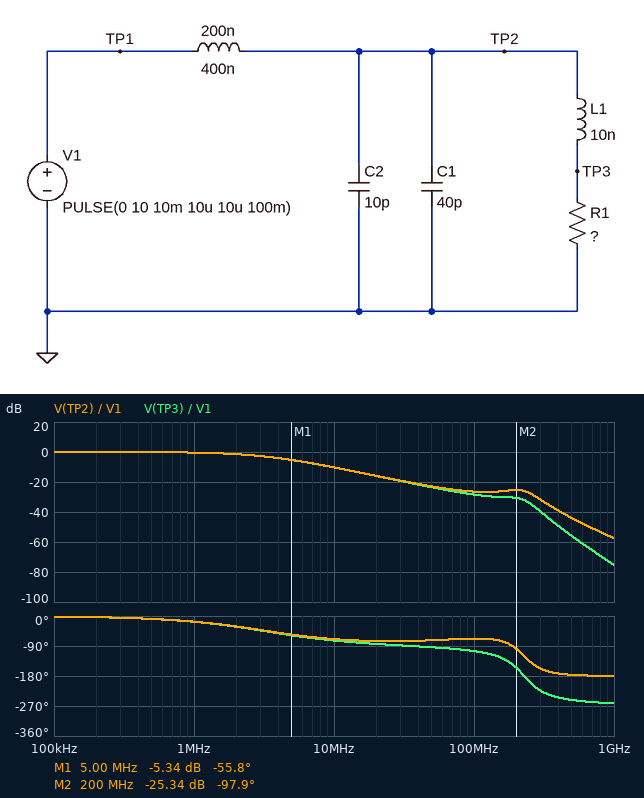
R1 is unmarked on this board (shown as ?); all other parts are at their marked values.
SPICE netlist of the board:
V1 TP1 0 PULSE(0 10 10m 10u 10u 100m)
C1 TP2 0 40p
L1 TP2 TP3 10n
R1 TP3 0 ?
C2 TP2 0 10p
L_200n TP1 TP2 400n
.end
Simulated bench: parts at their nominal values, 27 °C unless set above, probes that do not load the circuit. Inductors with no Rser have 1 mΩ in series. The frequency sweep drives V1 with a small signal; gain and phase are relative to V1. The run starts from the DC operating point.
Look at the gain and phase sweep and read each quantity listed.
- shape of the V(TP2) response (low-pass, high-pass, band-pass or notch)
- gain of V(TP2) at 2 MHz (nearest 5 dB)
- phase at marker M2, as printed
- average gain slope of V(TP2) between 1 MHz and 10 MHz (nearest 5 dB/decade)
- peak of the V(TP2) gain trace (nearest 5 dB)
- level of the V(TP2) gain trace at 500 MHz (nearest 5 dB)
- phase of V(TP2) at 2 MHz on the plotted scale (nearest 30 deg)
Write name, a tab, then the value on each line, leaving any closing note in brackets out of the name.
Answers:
shape of the V(TP2) response	low-pass
gain of V(TP2) at 2 MHz	0 dB
phase at marker M2, as printed	-97.9 deg
average gain slope of V(TP2) between 1 MHz and 10 MHz	-10 dB/decade
peak of the V(TP2) gain trace	0 dB
level of the V(TP2) gain trace at 500 MHz	-45 dB
phase of V(TP2) at 2 MHz on the plotted scale	-30 deg
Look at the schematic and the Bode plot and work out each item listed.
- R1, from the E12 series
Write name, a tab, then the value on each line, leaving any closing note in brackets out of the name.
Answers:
R1, from the E12 series	8.2 Ω
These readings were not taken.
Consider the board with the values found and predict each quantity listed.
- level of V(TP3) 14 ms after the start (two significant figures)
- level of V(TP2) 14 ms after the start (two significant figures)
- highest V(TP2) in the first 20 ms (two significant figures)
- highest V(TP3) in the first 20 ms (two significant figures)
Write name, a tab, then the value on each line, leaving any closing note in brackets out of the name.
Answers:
level of V(TP3) 14 ms after the start	10 V
level of V(TP2) 14 ms after the start	10 V
highest V(TP2) in the first 20 ms	10 V
highest V(TP3) in the first 20 ms	10 V
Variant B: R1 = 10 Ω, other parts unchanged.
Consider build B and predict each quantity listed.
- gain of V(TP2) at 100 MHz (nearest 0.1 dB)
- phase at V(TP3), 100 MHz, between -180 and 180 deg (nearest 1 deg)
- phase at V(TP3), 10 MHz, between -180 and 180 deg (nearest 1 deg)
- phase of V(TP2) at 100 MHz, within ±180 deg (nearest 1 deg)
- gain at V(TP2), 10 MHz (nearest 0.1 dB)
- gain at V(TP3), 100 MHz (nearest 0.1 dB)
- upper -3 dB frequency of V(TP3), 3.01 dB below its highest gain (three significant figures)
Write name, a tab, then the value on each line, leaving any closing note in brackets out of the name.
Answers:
gain of V(TP2) at 100 MHz	-25.4 dB
phase at V(TP3), 100 MHz, between -180 and 180 deg	-108 deg
phase at V(TP3), 10 MHz, between -180 and 180 deg	-70 deg
phase of V(TP2) at 100 MHz, within ±180 deg	-76 deg
gain at V(TP2), 10 MHz	-8.7 dB
gain at V(TP3), 100 MHz	-26.8 dB
upper -3 dB frequency of V(TP3), 3.01 dB below its highest gain	3.93 MHz
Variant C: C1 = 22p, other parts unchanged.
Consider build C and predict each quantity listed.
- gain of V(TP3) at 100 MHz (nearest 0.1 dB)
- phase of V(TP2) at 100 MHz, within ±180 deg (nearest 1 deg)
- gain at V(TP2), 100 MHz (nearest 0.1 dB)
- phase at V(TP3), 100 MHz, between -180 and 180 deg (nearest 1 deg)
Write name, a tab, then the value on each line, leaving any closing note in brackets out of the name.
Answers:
gain of V(TP3) at 100 MHz	-28.9 dB
phase of V(TP2) at 100 MHz, within ±180 deg	-61 deg
gain at V(TP2), 100 MHz	-26.9 dB
phase at V(TP3), 100 MHz, between -180 and 180 deg	-98 deg
